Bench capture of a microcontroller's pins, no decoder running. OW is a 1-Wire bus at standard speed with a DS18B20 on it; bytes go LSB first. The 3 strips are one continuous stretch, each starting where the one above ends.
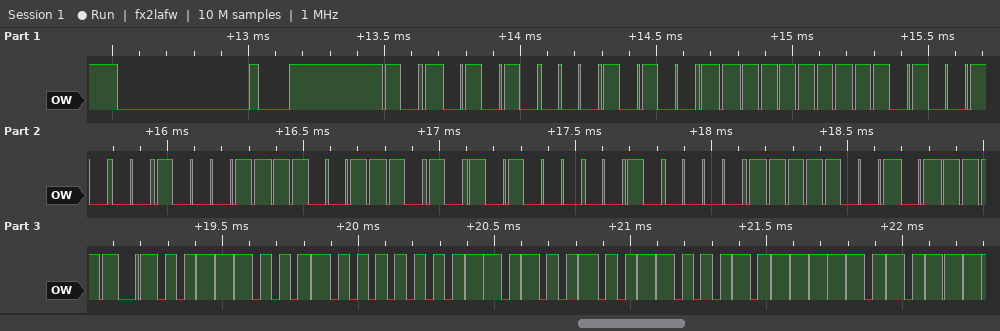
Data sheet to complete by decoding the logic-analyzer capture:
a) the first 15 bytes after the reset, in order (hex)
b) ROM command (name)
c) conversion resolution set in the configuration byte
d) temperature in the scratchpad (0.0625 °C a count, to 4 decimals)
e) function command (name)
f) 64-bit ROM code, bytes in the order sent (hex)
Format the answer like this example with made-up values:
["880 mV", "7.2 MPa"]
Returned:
["55 28 FF 4B C4 73 15 04 9F BE 1C 01 4B 46 5F", "Match ROM", "11 bits", "17.7500 °C", "Read Scratchpad", "28 FF 4B C4 73 15 04 9F"]
